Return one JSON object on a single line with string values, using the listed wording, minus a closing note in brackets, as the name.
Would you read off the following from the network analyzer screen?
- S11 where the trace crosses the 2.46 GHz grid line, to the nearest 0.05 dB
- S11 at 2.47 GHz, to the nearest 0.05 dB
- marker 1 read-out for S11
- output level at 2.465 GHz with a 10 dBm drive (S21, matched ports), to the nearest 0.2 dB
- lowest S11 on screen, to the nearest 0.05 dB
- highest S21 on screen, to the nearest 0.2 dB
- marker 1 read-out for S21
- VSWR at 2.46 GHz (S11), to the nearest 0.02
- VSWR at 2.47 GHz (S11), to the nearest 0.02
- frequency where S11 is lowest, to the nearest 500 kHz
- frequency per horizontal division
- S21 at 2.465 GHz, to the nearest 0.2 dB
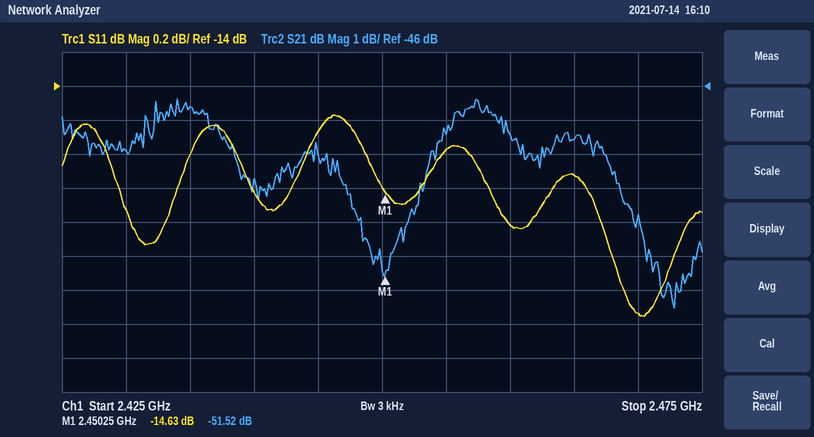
{"S11 where the trace crosses the 2.46 GHz grid line, to the nearest 0.05 dB": "-14.80 dB", "S11 at 2.47 GHz, to the nearest 0.05 dB": "-15.35 dB", "marker 1 read-out for S11": "-14.63 dB", "output level at 2.465 GHz with a 10 dBm drive (S21, matched ports), to the nearest 0.2 dB": "-37.6 dBm", "lowest S11 on screen, to the nearest 0.05 dB": "-15.35 dB", "highest S21 on screen, to the nearest 0.2 dB": "-46.4 dB", "marker 1 read-out for S21": "-51.52 dB", "VSWR at 2.46 GHz (S11), to the nearest 0.02": "1.44", "VSWR at 2.47 GHz (S11), to the nearest 0.02": "1.42", "frequency where S11 is lowest, to the nearest 500 kHz": "2.4705 GHz", "frequency per horizontal division": "5 MHz", "S21 at 2.465 GHz, to the nearest 0.2 dB": "-47.6 dB"}
